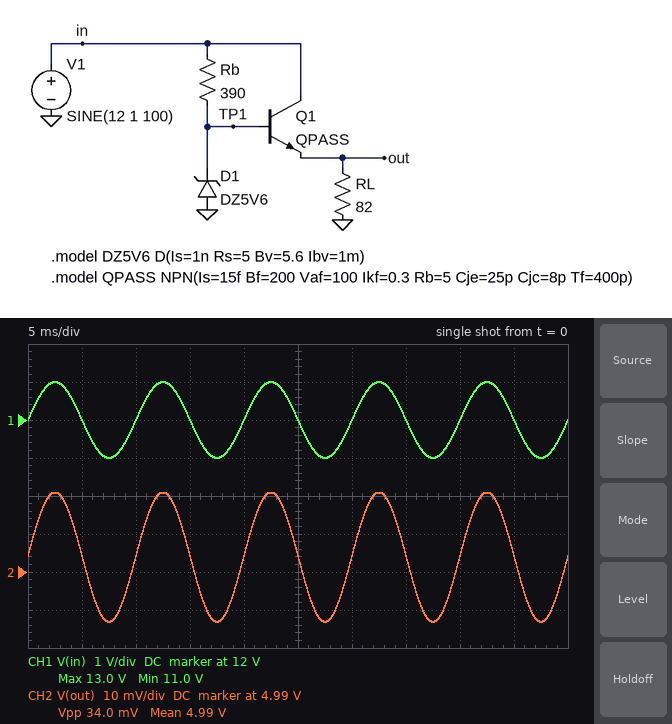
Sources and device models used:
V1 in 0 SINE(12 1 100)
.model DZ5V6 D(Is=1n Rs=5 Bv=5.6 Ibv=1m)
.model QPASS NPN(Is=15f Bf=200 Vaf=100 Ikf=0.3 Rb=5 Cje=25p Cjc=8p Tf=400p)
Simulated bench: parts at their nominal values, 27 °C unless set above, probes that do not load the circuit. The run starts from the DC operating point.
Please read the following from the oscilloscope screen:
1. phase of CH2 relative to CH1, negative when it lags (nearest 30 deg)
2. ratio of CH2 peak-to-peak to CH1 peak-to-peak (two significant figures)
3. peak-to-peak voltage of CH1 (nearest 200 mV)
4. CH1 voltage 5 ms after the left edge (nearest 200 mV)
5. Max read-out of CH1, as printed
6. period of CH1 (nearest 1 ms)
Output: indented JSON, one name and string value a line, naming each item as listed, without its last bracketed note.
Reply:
{
  "phase of CH2 relative to CH1, negative when it lags": "0 deg",
  "ratio of CH2 peak-to-peak to CH1 peak-to-peak": "0.017",
  "peak-to-peak voltage of CH1": "2.0 V",
  "CH1 voltage 5 ms after the left edge": "12.0 V",
  "Max read-out of CH1, as printed": "13.0 V",
  "period of CH1": "10 ms"
}
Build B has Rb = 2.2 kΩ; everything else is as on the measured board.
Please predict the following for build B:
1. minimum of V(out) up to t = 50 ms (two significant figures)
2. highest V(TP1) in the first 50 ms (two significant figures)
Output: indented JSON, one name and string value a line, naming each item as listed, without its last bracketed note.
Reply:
{
  "minimum of V(out) up to t = 50 ms": "4.9 V",
  "highest V(TP1) in the first 50 ms": "5.6 V"
}
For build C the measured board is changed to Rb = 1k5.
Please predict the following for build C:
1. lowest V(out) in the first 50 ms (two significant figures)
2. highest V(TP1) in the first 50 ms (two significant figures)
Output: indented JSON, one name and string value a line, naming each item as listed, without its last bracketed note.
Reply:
{
  "lowest V(out) in the first 50 ms": "4.9 V",
  "highest V(TP1) in the first 50 ms": "5.7 V"
}
